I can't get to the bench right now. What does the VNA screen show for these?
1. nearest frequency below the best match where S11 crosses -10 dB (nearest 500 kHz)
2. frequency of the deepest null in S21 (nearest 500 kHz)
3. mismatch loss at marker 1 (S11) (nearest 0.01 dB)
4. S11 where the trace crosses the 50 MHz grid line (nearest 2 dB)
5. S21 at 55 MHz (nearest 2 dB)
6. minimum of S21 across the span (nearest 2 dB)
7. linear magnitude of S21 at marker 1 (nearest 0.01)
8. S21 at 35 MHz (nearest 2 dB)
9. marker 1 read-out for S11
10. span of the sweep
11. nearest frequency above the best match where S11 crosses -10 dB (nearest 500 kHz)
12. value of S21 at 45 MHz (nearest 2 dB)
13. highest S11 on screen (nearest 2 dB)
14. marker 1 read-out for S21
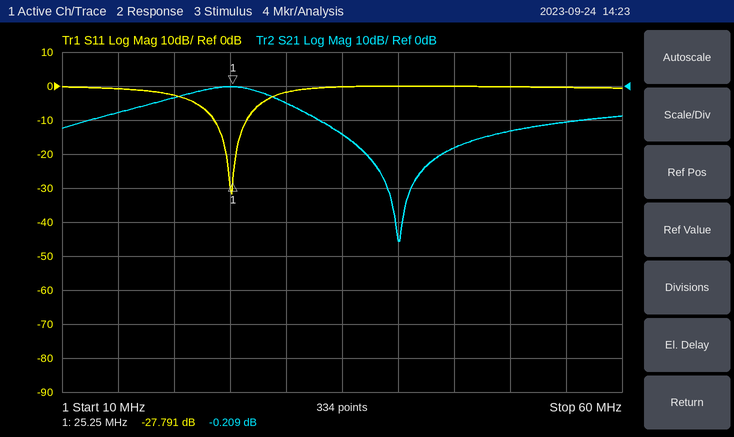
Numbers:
23.5 MHz
40.0 MHz
0.01 dB
0 dB
-10 dB
-46 dB
0.98
-14 dB
-27.791 dB
50 MHz
26.5 MHz
-18 dB
0 dB
-0.209 dB
